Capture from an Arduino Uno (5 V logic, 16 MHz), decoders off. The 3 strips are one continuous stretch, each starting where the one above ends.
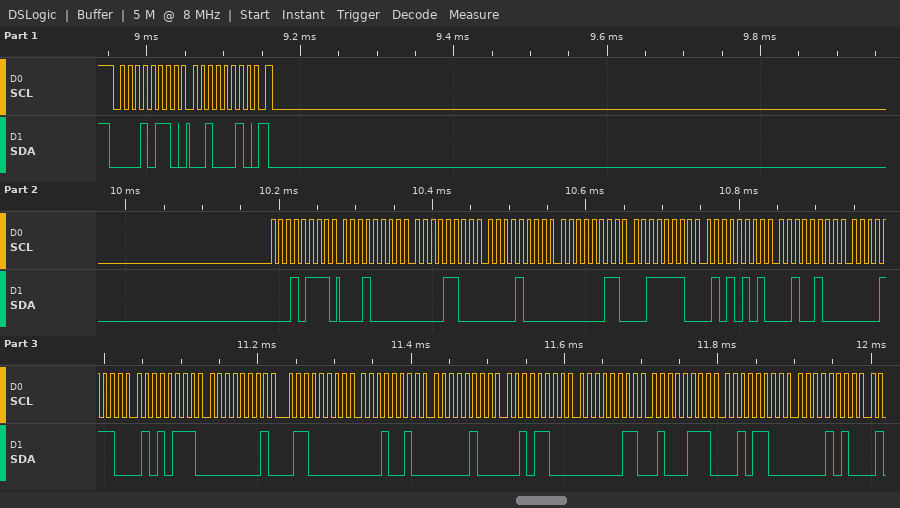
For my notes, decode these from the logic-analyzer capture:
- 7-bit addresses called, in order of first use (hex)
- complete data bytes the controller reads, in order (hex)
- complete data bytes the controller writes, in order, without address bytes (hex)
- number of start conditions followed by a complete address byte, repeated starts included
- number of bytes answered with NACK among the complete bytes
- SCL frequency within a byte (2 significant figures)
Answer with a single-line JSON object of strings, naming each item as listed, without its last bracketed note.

{"7-bit addresses called, in order of first use": "0x0B", "complete data bytes the controller reads, in order": "10 0C 08 03 3E 55 24 0E 57 01 60 12 04 2C 03 47 2C 0A", "complete data bytes the controller writes, in order, without address bytes": "22", "number of start conditions followed by a complete address byte, repeated starts included": "2", "number of bytes answered with NACK among the complete bytes": "0", "SCL frequency within a byte": "100 kHz"}
